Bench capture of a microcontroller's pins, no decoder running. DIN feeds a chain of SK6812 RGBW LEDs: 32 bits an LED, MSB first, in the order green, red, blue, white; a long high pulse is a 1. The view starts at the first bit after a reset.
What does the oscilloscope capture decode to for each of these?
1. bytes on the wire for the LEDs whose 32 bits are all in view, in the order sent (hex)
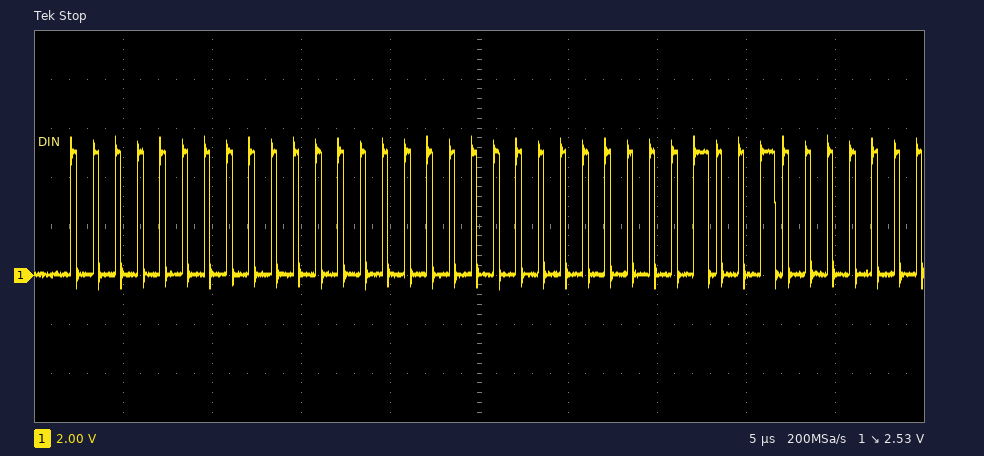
00 00 00 09
